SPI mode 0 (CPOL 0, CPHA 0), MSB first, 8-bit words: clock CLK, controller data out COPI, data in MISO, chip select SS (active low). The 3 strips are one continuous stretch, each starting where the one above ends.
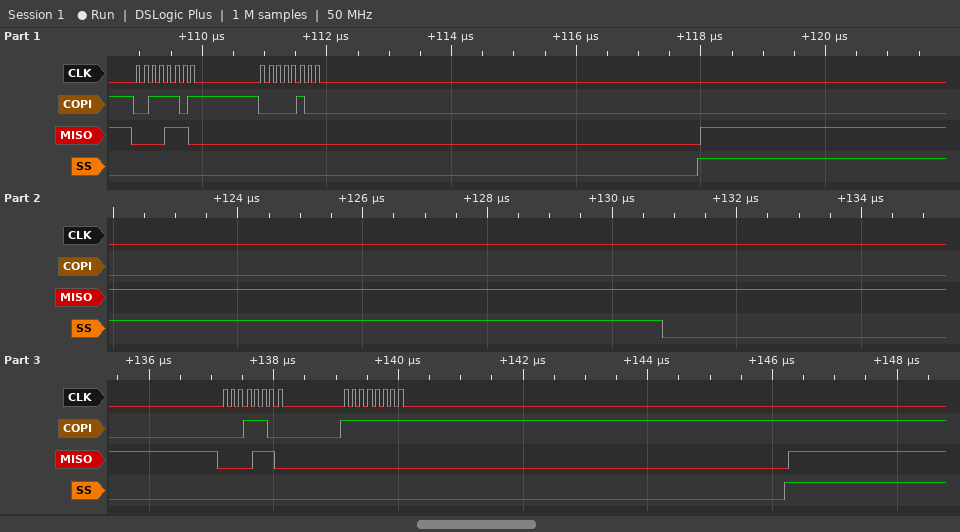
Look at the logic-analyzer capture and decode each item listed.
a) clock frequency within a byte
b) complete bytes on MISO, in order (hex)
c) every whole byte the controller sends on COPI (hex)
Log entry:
8 MHz
0E 00 0E 00
3D 04 1C FF
